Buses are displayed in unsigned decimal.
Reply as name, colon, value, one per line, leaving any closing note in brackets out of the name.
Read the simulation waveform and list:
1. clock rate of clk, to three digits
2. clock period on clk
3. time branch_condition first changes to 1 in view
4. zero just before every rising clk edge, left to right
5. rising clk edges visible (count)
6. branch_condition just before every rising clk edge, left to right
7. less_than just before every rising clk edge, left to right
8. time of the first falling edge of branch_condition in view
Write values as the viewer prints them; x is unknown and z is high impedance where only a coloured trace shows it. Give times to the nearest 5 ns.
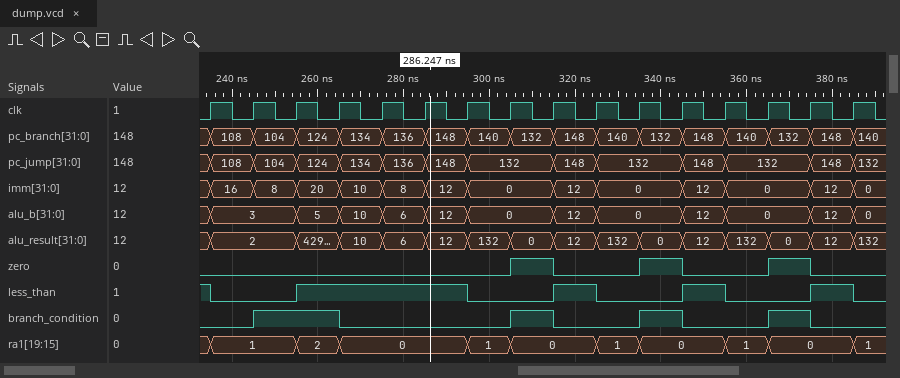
clock rate of clk, to three digits: 100 MHz
clock period on clk: 10 ns
time branch_condition first changes to 1 in view: 245 ns
zero just before every rising clk edge, left to right: 0 0 0 0 0 0 0 0 1 0 0 1 0 0 1 0
rising clk edges visible: 16
branch_condition just before every rising clk edge, left to right: 0 0 1 1 0 0 0 0 1 0 0 1 0 0 1 0
less_than just before every rising clk edge, left to right: 1 0 0 1 1 1 1 0 0 1 0 0 1 0 0 1
time of the first falling edge of branch_condition in view: 265 ns
